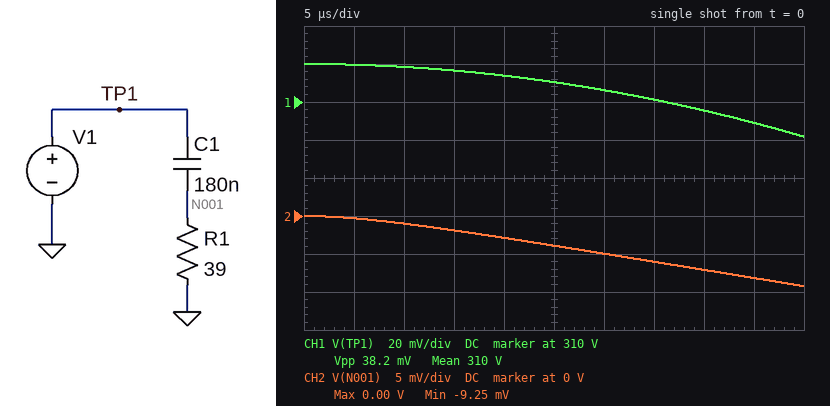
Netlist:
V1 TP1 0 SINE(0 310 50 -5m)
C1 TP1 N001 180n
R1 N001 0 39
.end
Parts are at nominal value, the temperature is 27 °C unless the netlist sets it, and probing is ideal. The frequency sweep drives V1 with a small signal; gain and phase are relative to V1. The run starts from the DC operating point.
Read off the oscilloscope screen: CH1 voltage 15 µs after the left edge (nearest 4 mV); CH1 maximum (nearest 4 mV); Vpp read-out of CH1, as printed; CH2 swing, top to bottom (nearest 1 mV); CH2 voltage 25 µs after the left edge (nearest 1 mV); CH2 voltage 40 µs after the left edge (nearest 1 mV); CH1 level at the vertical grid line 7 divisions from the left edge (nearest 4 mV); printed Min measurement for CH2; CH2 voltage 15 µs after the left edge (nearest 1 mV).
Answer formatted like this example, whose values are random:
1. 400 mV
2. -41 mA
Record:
1. 309.996 V
2. 310.000 V
3. 38.2 mV
4. 9 mV
5. -4 mV
6. -7 mV
7. 309.980 V
8. -9.25 mV
9. -2 mV
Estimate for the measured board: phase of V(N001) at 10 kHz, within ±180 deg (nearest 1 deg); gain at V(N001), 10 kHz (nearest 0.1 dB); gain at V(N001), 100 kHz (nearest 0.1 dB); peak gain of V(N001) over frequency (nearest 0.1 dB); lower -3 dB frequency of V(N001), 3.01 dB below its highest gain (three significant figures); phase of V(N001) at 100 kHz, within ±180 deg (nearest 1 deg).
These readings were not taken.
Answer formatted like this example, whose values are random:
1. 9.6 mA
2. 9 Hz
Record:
1. 66 deg
2. -7.9 dB
3. -0.2 dB
4. 0 dB
5. 22.7 kHz
6. 13 deg
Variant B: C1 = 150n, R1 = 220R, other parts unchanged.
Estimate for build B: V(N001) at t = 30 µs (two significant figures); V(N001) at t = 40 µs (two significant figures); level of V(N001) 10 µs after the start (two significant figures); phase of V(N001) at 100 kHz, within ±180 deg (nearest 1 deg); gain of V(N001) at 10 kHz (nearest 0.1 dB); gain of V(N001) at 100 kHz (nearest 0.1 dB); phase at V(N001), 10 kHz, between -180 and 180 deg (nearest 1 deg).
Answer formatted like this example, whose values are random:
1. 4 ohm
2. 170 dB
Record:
1. -10 mV
2. -17 mV
3. -1.4 mV
4. 3 deg
5. -0.9 dB
6. 0 dB
7. 26 deg
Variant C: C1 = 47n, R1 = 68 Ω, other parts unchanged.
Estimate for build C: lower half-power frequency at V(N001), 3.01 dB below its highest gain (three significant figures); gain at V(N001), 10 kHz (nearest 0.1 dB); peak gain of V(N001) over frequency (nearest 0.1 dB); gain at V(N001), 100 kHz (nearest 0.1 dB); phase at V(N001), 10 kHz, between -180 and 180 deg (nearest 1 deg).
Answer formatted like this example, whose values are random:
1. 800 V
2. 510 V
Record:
1. 49.8 kHz
2. -14.1 dB
3. 0 dB
4. -1.0 dB
5. 79 deg
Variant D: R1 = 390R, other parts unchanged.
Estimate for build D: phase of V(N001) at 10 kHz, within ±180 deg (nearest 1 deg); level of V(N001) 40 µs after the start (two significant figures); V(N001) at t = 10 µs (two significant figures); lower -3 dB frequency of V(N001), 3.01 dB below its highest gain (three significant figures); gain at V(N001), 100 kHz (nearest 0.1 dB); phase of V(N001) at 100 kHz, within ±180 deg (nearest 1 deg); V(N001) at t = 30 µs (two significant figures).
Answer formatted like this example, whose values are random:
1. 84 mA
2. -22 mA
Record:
1. 13 deg
2. -20 mV
3. -1.5 mV
4. 2.27 kHz
5. 0 dB
6. 1 deg
7. -12 mV
